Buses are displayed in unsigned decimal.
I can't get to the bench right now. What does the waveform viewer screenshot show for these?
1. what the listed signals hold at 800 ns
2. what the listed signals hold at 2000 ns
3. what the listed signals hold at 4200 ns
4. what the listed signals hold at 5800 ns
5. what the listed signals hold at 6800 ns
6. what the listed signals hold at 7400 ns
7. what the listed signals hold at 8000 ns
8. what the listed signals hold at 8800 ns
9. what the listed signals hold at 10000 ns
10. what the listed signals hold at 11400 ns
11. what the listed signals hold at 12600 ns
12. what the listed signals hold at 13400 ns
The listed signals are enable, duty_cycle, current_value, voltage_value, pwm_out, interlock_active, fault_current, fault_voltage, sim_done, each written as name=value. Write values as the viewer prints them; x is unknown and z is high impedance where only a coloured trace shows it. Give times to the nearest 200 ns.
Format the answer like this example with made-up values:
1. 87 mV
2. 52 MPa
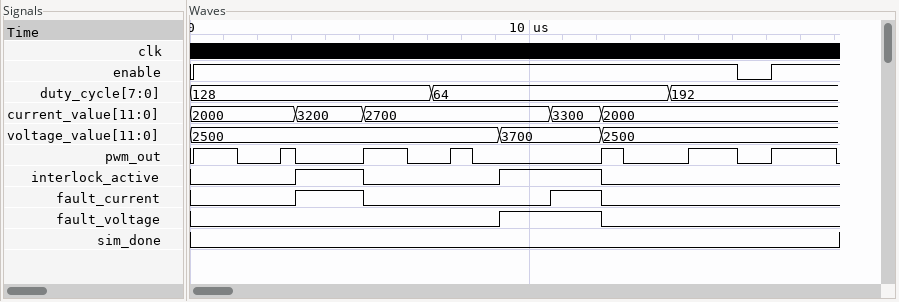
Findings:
1. enable=1, duty_cycle=128, current_value=2000, voltage_value=2500, pwm_out=1, interlock_active=0, fault_current=0, fault_voltage=0, sim_done=0
2. enable=1, duty_cycle=128, current_value=2000, voltage_value=2500, pwm_out=0, interlock_active=0, fault_current=0, fault_voltage=0, sim_done=0
3. enable=1, duty_cycle=128, current_value=3200, voltage_value=2500, pwm_out=0, interlock_active=1, fault_current=1, fault_voltage=0, sim_done=0
4. enable=1, duty_cycle=128, current_value=2700, voltage_value=2500, pwm_out=1, interlock_active=0, fault_current=0, fault_voltage=0, sim_done=0
5. enable=1, duty_cycle=128, current_value=2700, voltage_value=2500, pwm_out=0, interlock_active=0, fault_current=0, fault_voltage=0, sim_done=0
6. enable=1, duty_cycle=64, current_value=2700, voltage_value=2500, pwm_out=0, interlock_active=0, fault_current=0, fault_voltage=0, sim_done=0
7. enable=1, duty_cycle=64, current_value=2700, voltage_value=2500, pwm_out=1, interlock_active=0, fault_current=0, fault_voltage=0, sim_done=0
8. enable=1, duty_cycle=64, current_value=2700, voltage_value=2500, pwm_out=0, interlock_active=0, fault_current=0, fault_voltage=0, sim_done=0
9. enable=1, duty_cycle=64, current_value=2700, voltage_value=3700, pwm_out=0, interlock_active=1, fault_current=0, fault_voltage=1, sim_done=0
10. enable=1, duty_cycle=64, current_value=3300, voltage_value=3700, pwm_out=0, interlock_active=1, fault_current=1, fault_voltage=1, sim_done=0
11. enable=1, duty_cycle=64, current_value=2000, voltage_value=2500, pwm_out=1, interlock_active=0, fault_current=0, fault_voltage=0, sim_done=0
12. enable=1, duty_cycle=64, current_value=2000, voltage_value=2500, pwm_out=0, interlock_active=0, fault_current=0, fault_voltage=0, sim_done=0
